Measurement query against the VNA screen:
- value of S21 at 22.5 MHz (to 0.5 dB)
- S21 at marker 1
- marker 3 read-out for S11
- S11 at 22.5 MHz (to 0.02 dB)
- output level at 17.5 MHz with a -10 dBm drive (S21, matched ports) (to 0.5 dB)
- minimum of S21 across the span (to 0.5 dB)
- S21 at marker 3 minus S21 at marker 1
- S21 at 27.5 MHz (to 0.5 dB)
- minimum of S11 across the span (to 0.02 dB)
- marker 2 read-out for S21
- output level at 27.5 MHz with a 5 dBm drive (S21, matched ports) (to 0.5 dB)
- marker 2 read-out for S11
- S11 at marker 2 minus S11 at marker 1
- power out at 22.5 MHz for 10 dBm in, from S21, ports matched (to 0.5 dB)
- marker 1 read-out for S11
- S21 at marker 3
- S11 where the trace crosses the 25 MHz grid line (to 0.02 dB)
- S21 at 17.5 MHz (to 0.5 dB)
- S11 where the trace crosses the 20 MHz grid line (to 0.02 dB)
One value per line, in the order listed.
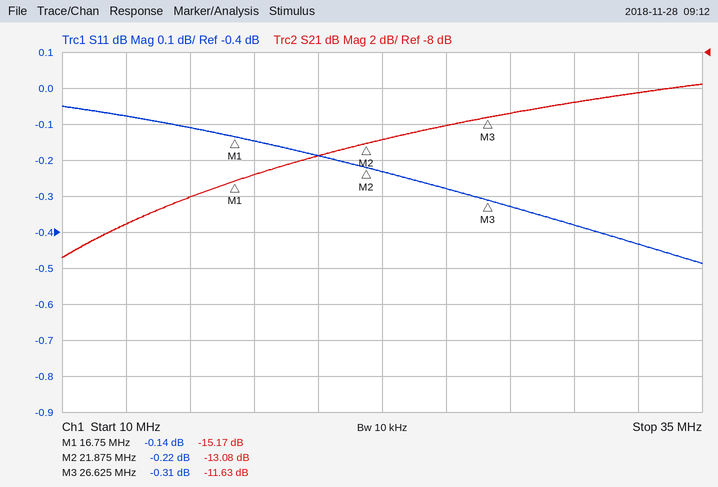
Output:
-13.0 dB
-15.17 dB
-0.31 dB
-0.24 dB
-25.0 dBm
-19.5 dB
3.54 dB
-11.5 dB
-0.48 dB
-13.08 dB
-6.5 dBm
-0.22 dB
-0.08 dB
-3.0 dBm
-0.14 dB
-11.63 dB
-0.28 dB
-15.0 dB
-0.18 dB
